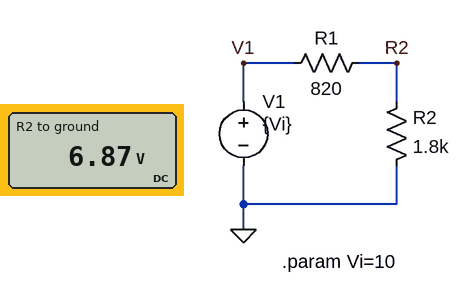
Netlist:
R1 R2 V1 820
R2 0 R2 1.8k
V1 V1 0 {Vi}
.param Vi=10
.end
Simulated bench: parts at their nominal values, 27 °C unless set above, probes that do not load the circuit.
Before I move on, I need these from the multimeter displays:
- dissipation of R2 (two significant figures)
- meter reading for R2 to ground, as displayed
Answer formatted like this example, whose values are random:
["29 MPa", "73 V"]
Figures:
["26 mW", "6.87 V"]
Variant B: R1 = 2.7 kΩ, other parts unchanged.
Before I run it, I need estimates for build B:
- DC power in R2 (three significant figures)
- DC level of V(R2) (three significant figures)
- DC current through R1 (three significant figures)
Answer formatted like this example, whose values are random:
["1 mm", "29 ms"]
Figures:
["8.89 mW", "4.00 V", "2.22 mA"]
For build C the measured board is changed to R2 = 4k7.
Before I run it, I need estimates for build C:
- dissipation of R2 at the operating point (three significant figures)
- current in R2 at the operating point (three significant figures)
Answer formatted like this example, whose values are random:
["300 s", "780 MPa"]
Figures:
["15.4 mW", "1.81 mA"]
